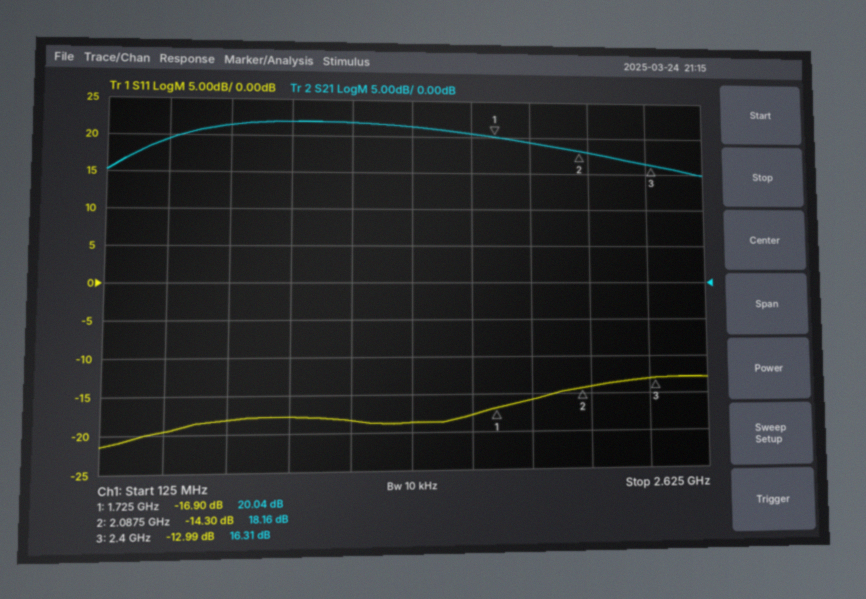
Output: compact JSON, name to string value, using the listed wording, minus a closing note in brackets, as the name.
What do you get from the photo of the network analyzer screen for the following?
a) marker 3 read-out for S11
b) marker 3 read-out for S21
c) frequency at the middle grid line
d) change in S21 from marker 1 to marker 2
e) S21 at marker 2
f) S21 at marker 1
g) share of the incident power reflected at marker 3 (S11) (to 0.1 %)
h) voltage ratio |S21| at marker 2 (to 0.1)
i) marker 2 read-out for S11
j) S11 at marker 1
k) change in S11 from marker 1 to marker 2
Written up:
{"marker 3 read-out for S11": "-12.99 dB", "marker 3 read-out for S21": "16.31 dB", "frequency at the middle grid line": "1.375 GHz", "change in S21 from marker 1 to marker 2": "-1.88 dB", "S21 at marker 2": "18.16 dB", "S21 at marker 1": "20.04 dB", "share of the incident power reflected at marker 3 (S11)": "5.0 %", "voltage ratio |S21| at marker 2": "8.1", "marker 2 read-out for S11": "-14.30 dB", "S11 at marker 1": "-16.90 dB", "change in S11 from marker 1 to marker 2": "2.60 dB"}
